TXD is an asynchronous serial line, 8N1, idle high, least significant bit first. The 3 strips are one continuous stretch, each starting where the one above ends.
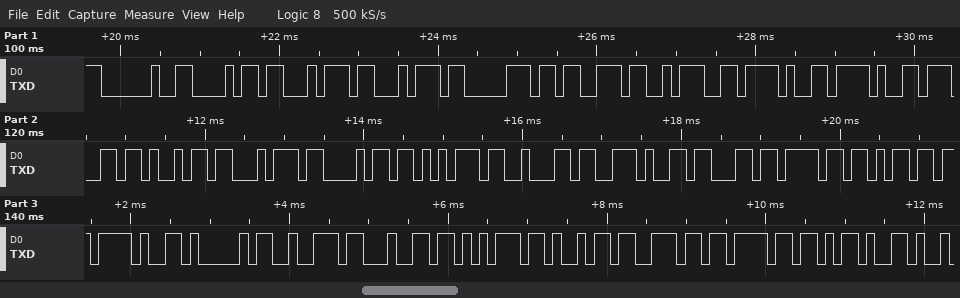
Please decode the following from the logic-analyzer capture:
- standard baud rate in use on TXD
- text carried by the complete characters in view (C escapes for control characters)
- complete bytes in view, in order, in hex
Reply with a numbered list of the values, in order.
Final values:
1. 9600 baud
2. " https://github.com/Arduino-"
3. 0x20 0x68 0x74 0x74 0x70 0x73 0x3A 0x2F 0x2F 0x67 0x69 0x74 0x68 0x75 0x62 0x2E 0x63 0x6F 0x6D 0x2F 0x41 0x72 0x64 0x75 0x69 0x6E 0x6F 0x2D
